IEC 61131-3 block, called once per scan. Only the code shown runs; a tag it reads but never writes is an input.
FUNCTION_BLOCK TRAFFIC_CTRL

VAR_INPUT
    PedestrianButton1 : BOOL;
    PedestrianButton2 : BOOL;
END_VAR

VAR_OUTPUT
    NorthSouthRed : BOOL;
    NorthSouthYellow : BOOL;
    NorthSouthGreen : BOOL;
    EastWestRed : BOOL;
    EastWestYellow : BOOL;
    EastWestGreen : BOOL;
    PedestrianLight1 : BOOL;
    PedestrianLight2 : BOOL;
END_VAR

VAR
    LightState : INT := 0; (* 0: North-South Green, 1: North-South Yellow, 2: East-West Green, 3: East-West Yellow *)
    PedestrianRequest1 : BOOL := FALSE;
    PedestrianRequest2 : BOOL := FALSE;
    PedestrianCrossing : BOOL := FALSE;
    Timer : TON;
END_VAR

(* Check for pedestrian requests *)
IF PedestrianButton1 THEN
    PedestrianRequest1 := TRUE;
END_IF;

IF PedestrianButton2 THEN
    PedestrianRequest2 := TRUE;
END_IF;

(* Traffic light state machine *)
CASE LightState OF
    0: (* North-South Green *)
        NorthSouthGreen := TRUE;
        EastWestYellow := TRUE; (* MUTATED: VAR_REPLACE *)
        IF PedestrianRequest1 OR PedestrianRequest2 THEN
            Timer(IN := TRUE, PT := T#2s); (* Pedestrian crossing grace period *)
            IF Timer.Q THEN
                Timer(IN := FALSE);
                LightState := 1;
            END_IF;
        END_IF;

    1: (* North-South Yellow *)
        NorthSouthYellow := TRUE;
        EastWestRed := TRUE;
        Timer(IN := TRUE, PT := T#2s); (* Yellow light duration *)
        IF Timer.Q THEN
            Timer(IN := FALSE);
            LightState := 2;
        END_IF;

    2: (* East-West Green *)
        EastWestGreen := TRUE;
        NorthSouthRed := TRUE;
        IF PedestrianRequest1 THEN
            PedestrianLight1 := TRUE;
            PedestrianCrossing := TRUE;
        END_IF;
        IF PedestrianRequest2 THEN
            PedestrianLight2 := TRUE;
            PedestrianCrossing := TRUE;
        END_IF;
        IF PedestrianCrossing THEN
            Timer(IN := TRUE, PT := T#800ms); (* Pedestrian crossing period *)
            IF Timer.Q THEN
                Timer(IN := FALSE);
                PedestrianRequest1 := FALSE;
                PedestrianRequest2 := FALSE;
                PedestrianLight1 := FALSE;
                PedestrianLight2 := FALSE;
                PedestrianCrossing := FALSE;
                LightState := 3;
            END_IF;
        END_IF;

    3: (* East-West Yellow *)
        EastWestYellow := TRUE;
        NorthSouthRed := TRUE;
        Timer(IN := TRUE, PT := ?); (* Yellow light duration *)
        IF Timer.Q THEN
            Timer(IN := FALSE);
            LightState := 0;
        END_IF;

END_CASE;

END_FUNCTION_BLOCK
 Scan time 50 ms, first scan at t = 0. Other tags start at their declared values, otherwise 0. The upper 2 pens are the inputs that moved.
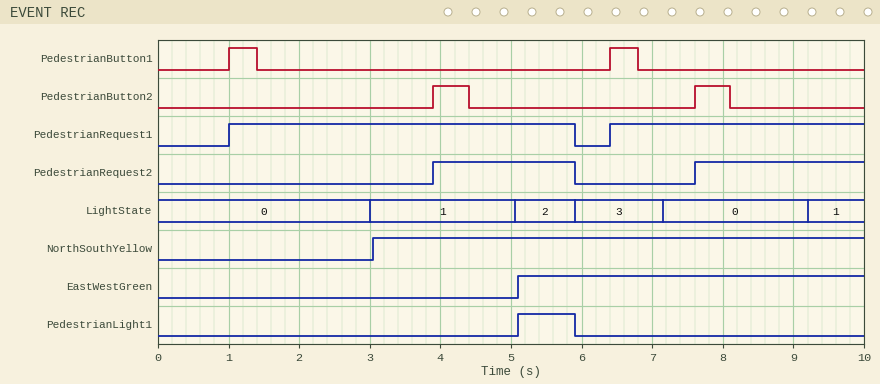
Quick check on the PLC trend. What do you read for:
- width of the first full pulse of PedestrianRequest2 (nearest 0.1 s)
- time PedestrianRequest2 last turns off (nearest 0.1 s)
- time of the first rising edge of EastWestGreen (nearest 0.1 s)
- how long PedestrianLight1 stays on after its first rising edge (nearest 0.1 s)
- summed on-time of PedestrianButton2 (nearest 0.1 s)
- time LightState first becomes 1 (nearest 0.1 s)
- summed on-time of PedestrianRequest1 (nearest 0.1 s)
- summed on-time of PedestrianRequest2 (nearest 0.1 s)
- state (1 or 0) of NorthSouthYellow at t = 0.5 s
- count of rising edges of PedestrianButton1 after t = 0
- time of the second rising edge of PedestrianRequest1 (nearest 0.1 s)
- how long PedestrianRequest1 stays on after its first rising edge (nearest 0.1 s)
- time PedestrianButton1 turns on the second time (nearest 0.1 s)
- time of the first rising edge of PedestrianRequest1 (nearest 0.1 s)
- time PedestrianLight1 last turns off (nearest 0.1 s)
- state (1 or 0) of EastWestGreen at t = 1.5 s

2.0 s
5.9 s
5.1 s
0.8 s
1.0 s
3.0 s
8.5 s
4.4 s
0
2
6.4 s
4.9 s
6.4 s
1.0 s
5.9 s
0
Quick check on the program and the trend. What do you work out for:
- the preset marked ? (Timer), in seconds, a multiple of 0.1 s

1.2 s
